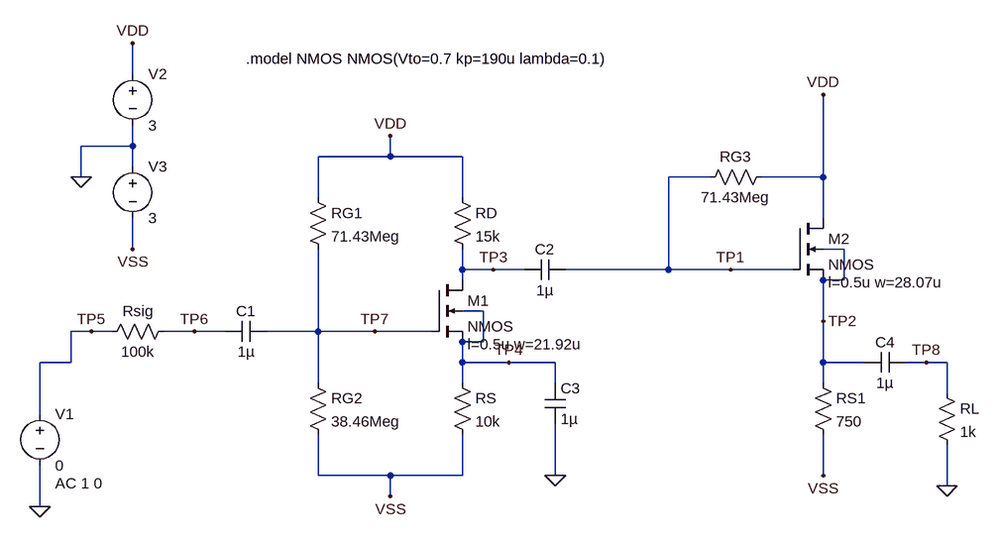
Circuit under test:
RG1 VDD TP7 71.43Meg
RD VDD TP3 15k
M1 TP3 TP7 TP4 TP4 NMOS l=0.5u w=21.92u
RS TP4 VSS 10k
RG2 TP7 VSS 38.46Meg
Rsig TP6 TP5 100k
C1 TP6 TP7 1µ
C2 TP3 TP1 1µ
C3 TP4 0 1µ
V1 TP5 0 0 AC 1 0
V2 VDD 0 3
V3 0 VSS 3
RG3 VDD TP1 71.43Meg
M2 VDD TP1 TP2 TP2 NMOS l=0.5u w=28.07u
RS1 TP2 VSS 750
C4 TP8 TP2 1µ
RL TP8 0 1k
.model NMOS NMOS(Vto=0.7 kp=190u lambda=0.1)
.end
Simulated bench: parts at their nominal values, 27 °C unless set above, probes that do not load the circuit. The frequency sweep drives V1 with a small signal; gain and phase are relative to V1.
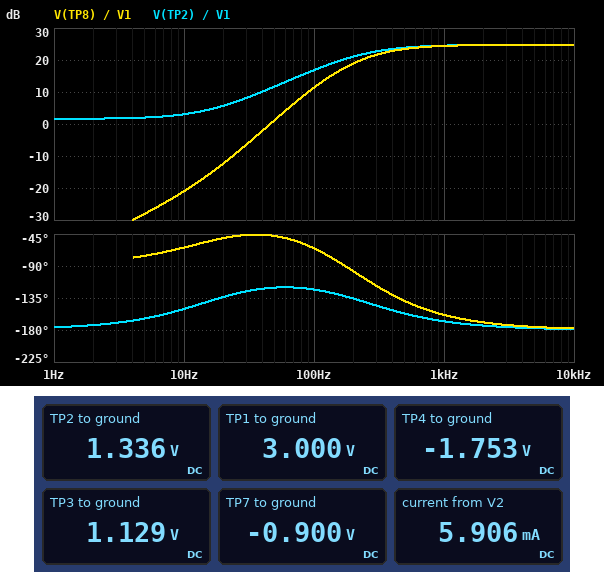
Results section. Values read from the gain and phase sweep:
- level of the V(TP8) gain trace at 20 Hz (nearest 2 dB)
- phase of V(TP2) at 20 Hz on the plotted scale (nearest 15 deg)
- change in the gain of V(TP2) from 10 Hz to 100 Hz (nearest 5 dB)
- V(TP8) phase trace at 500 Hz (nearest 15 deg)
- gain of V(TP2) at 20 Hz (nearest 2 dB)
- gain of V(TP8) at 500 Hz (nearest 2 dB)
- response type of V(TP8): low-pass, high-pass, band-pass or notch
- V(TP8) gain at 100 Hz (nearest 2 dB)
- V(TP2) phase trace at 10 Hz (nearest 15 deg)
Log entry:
-12 dB
-135 deg
15 dB
-135 deg
6 dB
24 dB
high-pass
12 dB
-150 deg
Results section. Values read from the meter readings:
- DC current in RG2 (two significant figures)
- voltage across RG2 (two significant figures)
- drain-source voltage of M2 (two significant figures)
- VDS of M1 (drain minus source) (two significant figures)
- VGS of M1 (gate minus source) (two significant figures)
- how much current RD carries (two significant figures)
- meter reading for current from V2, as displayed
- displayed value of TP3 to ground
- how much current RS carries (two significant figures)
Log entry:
55 nA
2.1 V
1.7 V
2.9 V
850 mV
120 µA
5.906 mA
1.129 V
120 µA
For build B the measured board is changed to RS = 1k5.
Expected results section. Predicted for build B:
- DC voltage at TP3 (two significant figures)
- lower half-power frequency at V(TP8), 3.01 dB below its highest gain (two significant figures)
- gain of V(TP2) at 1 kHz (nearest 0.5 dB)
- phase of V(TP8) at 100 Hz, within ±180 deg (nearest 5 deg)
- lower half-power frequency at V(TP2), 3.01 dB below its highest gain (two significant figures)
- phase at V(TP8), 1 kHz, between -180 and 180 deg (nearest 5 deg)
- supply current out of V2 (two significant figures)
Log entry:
-2.4 V
160 Hz
-26.0 dB
-120 deg
7.5 mHz
-170 deg
6.1 mA
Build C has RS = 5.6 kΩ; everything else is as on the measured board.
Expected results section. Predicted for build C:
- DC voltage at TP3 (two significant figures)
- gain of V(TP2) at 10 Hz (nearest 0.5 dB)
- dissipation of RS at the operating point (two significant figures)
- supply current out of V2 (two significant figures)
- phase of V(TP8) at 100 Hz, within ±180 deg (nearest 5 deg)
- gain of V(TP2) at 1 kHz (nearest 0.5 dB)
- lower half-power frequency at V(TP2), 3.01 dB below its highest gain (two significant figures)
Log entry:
-190 mV
7.0 dB
250 µW
6.0 mA
-70 deg
25.5 dB
270 Hz
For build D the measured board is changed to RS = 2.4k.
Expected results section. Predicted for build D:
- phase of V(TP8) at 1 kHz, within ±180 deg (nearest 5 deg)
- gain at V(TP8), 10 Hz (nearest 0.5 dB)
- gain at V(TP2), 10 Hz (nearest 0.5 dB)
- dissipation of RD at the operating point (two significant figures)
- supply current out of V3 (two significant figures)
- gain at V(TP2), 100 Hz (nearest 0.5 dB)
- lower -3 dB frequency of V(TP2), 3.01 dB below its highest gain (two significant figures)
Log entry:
-170 deg
-43.5 dB
-19.5 dB
1.7 mW
6.1 mA
-19.0 dB
8.7 mHz
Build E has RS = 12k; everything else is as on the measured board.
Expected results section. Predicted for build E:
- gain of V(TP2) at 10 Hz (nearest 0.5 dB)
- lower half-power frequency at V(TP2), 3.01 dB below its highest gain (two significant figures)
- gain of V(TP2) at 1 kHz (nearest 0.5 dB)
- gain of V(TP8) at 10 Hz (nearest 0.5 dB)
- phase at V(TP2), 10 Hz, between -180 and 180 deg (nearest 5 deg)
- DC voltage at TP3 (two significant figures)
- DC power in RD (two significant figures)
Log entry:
2.0 dB
220 Hz
24.0 dB
-22.0 dB
-145 deg
1.4 V
170 µW
